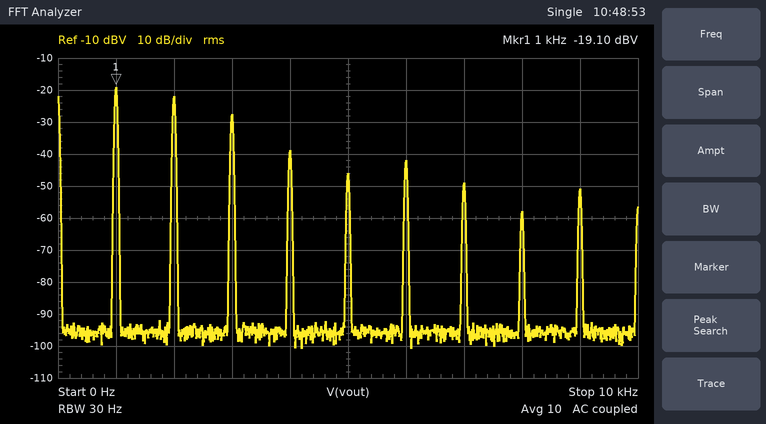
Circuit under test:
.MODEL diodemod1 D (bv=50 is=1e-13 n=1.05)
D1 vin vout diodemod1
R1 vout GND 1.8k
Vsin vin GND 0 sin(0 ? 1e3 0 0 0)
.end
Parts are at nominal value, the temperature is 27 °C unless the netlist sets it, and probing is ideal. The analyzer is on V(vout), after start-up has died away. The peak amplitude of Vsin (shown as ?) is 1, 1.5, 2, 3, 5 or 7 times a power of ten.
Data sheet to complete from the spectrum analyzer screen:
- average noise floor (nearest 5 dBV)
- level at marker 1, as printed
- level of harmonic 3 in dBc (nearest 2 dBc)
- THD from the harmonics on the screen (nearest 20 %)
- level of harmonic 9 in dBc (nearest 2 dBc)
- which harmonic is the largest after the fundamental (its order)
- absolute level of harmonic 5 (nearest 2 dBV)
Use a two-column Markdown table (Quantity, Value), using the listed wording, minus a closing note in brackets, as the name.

| Quantity | Value |
|---|---|
| average noise floor | -95 dBV |
| level at marker 1, as printed | -19.10 dBV |
| level of harmonic 3 in dBc | -8 dBc |
| THD from the harmonics on the screen | 80 % |
| level of harmonic 9 in dBc | -32 dBc |
| which harmonic is the largest after the fundamental | 2 |
| absolute level of harmonic 5 | -46 dBV |
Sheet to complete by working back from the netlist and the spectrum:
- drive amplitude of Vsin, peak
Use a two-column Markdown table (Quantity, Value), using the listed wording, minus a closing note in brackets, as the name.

| Quantity | Value |
|---|---|
| drive amplitude of Vsin, peak | 1 V |
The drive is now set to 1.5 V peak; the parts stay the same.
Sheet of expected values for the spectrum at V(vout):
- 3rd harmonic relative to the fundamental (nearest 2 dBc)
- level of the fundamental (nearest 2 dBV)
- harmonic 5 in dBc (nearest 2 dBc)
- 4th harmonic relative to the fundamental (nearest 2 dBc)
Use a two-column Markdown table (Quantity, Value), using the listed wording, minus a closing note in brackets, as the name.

| Quantity | Value |
|---|---|
| 3rd harmonic relative to the fundamental | -12 dBc |
| level of the fundamental | -12 dBV |
| harmonic 5 in dBc | -22 dBc |
| 4th harmonic relative to the fundamental | -34 dBc |
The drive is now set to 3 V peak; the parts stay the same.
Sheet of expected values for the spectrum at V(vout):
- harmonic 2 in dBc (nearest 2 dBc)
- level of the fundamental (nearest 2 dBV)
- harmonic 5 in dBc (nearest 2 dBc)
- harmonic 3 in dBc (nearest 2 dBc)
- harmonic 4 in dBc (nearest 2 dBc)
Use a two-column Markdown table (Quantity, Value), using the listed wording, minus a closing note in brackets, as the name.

| Quantity | Value |
|---|---|
| harmonic 2 in dBc | -6 dBc |
| level of the fundamental | -2 dBV |
| harmonic 5 in dBc | -26 dBc |
| harmonic 3 in dBc | -20 dBc |
| harmonic 4 in dBc | -22 dBc |
